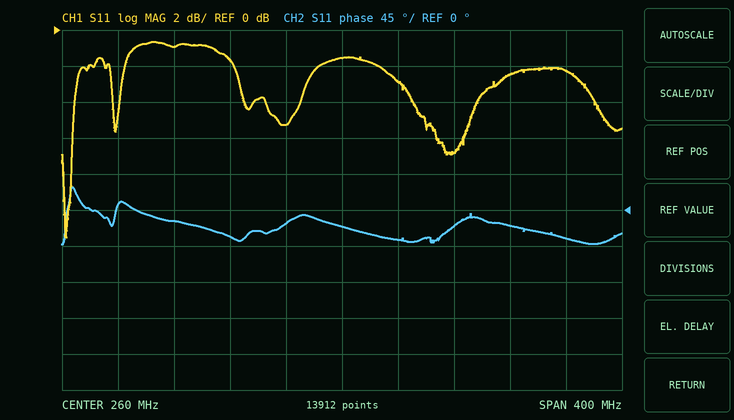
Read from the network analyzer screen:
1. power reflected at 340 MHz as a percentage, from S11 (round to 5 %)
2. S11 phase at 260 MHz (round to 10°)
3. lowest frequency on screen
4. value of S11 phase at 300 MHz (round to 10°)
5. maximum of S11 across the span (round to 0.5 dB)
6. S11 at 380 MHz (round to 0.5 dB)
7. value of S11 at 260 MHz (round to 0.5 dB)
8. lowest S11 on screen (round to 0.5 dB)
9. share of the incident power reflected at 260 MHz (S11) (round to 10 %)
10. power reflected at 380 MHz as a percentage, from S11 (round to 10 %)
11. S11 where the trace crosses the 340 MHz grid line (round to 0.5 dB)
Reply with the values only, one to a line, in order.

20 %
-20°
60 MHz
-40°
-0.5 dB
-2.5 dB
-1.5 dB
-11.5 dB
70 %
60 %
-7.0 dB
